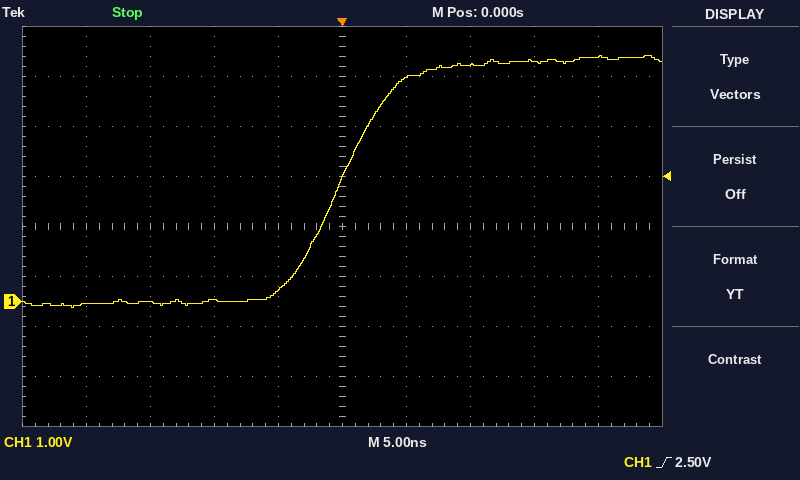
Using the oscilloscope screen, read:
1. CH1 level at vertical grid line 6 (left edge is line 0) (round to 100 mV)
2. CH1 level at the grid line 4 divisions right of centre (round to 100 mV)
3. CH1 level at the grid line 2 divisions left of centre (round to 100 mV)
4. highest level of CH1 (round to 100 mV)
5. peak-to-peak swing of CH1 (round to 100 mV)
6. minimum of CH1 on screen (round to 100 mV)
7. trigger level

4.5 V
4.9 V
0.0 V
4.9 V
5.0 V
-100 mV
2.50 V
